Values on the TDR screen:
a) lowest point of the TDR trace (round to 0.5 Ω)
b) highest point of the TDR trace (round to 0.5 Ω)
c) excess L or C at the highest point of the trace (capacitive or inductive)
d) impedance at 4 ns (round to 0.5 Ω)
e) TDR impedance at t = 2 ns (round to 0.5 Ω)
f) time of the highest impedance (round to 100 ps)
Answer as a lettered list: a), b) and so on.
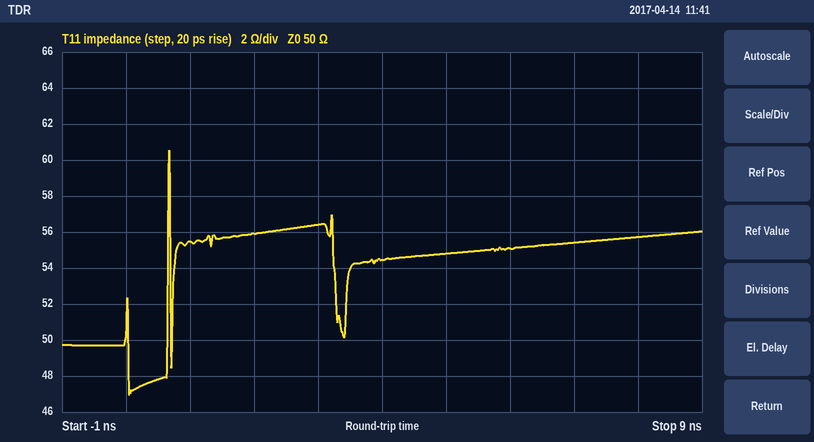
a) 47.0 Ω
b) 60.5 Ω
c) inductive
d) 54.5 Ω
e) 56.0 Ω
f) 700 ps
